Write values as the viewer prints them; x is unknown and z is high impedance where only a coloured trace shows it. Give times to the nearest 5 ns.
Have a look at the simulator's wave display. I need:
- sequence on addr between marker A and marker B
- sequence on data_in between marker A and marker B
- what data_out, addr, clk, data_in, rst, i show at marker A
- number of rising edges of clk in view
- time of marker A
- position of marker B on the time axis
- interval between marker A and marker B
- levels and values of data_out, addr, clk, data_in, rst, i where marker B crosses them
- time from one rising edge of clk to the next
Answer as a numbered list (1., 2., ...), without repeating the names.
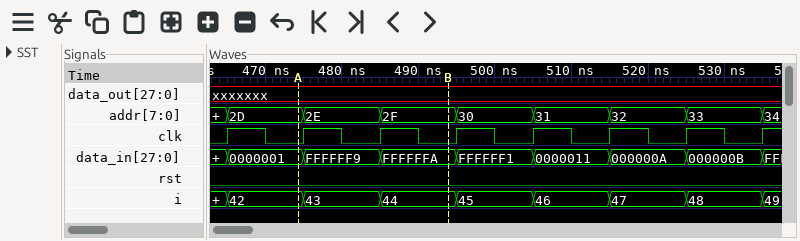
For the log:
1. 2D, 2E, 2F
2. 0000001, FFFFFF9, FFFFFFA
3. data_out=xxxxxxx, addr=2D, clk=0, data_in=0000001, rst=0, i=42
4. 8
5. 475 ns
6. 495 ns
7. 20 ns
8. data_out=xxxxxxx, addr=2F, clk=0, data_in=FFFFFFA, rst=0, i=44
9. 10 ns
